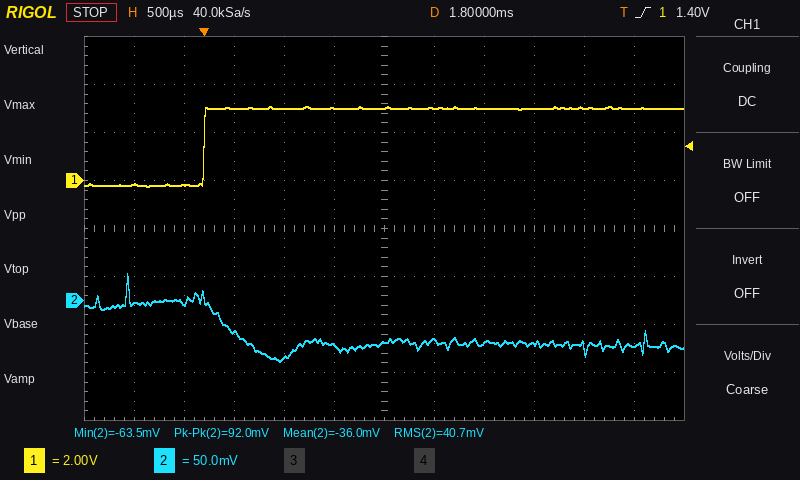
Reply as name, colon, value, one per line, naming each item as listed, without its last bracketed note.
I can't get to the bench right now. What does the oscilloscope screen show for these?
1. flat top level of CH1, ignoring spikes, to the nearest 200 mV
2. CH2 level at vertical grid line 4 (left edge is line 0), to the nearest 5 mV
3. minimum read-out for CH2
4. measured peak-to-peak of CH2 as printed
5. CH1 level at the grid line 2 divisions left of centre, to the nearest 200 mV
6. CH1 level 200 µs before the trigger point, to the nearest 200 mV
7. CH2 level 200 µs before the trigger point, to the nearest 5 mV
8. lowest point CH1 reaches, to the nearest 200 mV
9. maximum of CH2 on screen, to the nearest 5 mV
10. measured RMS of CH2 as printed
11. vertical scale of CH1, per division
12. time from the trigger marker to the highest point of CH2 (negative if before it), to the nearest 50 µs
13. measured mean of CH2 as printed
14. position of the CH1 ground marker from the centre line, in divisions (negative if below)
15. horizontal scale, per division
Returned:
flat top level of CH1, ignoring spikes, to the nearest 200 mV: 3.0 V
CH2 level at vertical grid line 4 (left edge is line 0), to the nearest 5 mV: -60 mV
minimum read-out for CH2: -63.5 mV
measured peak-to-peak of CH2 as printed: 92.0 mV
CH1 level at the grid line 2 divisions left of centre, to the nearest 200 mV: 3.0 V
CH1 level 200 µs before the trigger point, to the nearest 200 mV: -200 mV
CH2 level 200 µs before the trigger point, to the nearest 5 mV: 0 mV
lowest point CH1 reaches, to the nearest 200 mV: -200 mV
maximum of CH2 on screen, to the nearest 5 mV: 30 mV
measured RMS of CH2 as printed: 40.7 mV
vertical scale of CH1, per division: 2 V
time from the trigger marker to the highest point of CH2 (negative if before it), to the nearest 50 µs: -750 µs
measured mean of CH2 as printed: -36.0 mV
position of the CH1 ground marker from the centre line, in divisions: +1.0 div
horizontal scale, per division: 500 µs
